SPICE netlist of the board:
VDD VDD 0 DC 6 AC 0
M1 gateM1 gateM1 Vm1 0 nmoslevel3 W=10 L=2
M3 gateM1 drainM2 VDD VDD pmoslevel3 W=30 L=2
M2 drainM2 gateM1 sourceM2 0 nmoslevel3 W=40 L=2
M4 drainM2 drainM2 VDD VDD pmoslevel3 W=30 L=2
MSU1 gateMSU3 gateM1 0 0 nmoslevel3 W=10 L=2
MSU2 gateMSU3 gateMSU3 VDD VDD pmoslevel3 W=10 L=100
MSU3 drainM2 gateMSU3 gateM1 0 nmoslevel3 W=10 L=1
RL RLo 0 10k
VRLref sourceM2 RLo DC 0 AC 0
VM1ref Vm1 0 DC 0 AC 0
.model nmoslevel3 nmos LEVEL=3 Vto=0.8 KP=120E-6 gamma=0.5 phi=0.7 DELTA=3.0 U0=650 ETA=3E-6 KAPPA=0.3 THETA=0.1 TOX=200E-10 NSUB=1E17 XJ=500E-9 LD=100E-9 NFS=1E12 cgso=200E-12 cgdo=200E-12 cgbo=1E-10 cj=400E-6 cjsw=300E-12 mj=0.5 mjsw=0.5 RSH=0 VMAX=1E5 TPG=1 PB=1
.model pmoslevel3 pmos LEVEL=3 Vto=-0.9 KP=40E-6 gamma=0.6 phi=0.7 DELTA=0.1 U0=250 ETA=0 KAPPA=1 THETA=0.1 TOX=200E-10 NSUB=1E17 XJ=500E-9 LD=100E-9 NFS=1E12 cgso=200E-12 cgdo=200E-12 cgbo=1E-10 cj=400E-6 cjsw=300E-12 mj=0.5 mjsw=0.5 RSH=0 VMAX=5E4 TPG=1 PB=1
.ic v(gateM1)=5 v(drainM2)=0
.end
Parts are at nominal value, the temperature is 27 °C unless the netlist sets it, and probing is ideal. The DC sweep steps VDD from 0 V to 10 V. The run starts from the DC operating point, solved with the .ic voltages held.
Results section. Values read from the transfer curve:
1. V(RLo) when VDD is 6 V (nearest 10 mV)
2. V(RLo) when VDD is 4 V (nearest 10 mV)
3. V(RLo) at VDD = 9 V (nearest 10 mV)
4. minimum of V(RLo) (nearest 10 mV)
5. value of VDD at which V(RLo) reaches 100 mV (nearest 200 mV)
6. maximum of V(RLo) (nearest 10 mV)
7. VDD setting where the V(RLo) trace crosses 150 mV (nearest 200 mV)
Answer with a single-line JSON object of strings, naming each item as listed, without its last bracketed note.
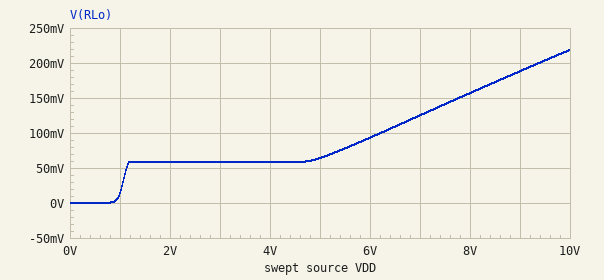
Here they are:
{"V(RLo) when VDD is 6 V": "90 mV", "V(RLo) when VDD is 4 V": "60 mV", "V(RLo) at VDD = 9 V": "190 mV", "minimum of V(RLo)": "0 V", "value of VDD at which V(RLo) reaches 100 mV": "6.2 V", "maximum of V(RLo)": "220 mV", "VDD setting where the V(RLo) trace crosses 150 mV": "7.8 V"}
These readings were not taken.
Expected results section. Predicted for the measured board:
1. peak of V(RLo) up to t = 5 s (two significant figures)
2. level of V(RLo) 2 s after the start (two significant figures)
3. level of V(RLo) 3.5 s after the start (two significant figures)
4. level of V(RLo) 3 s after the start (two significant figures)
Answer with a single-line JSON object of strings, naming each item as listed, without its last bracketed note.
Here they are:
{"peak of V(RLo) up to t = 5 s": "44 mV", "level of V(RLo) 2 s after the start": "14 mV", "level of V(RLo) 3.5 s after the start": "28 mV", "level of V(RLo) 3 s after the start": "23 mV"}
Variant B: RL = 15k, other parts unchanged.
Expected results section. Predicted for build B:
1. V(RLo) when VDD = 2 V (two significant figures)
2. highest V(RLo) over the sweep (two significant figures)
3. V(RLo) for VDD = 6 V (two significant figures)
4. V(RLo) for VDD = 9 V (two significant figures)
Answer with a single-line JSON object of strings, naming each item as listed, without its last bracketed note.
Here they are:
{"V(RLo) when VDD = 2 V": "45 mV", "highest V(RLo) over the sweep": "240 mV", "V(RLo) for VDD = 6 V": "100 mV", "V(RLo) for VDD = 9 V": "200 mV"}
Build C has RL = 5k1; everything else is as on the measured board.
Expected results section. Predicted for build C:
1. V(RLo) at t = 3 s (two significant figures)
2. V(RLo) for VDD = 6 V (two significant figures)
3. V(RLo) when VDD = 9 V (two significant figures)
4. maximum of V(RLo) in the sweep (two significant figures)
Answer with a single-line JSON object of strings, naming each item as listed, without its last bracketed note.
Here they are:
{"V(RLo) at t = 3 s": "23 mV", "V(RLo) for VDD = 6 V": "120 mV", "V(RLo) when VDD = 9 V": "160 mV", "maximum of V(RLo) in the sweep": "190 mV"}
